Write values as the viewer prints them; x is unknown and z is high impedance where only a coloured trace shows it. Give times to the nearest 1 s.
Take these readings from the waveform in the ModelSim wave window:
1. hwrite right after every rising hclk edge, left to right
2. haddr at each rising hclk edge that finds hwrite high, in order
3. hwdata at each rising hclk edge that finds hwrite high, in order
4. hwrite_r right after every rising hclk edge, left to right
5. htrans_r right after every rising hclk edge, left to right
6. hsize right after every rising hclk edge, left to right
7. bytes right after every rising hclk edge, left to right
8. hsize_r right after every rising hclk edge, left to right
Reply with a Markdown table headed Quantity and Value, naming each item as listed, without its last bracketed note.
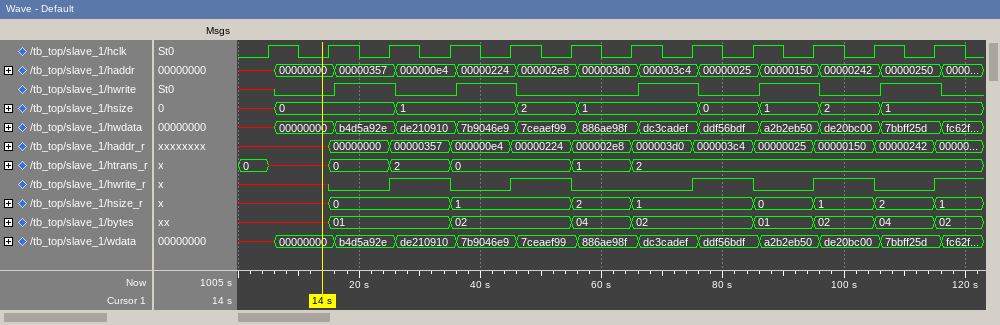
| Quantity | Value |
|---|---|
| hwrite right after every rising hclk edge, left to right | x 0 1 0 1 0 0 1 0 1 0 1 |
| haddr at each rising hclk edge that finds hwrite high, in order | 00000357, 00000224, 000003c4, 00000150, 00000250 |
| hwdata at each rising hclk edge that finds hwrite high, in order | b4d5a92e, 7b9046e9, dc3cadef, a2b2eb50, 7bbff25d |
| hwrite_r right after every rising hclk edge, left to right | x 0 1 0 1 0 0 1 0 1 0 1 |
| htrans_r right after every rising hclk edge, left to right | x, 0, 2, 0, 0, 1, 2, 2, 2, 2, 2, 2 |
| hsize right after every rising hclk edge, left to right | x, 0, 0, 1, 1, 2, 1, 1, 0, 1, 2, 1 |
| bytes right after every rising hclk edge, left to right | x, 01, 01, 02, 02, 04, 02, 02, 01, 02, 04, 02 |
| hsize_r right after every rising hclk edge, left to right | x, 0, 0, 1, 1, 2, 1, 1, 0, 1, 2, 1 |
